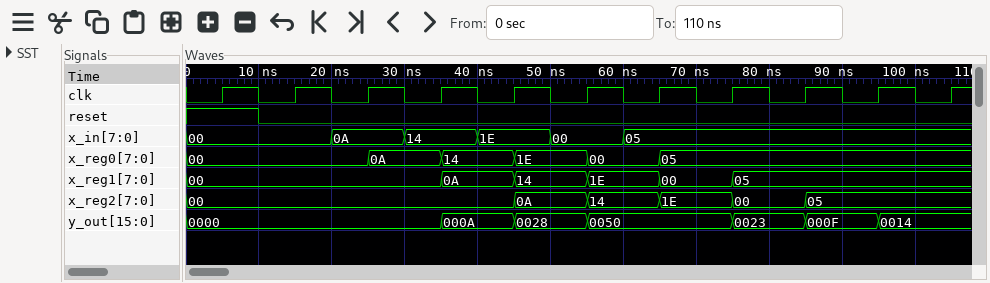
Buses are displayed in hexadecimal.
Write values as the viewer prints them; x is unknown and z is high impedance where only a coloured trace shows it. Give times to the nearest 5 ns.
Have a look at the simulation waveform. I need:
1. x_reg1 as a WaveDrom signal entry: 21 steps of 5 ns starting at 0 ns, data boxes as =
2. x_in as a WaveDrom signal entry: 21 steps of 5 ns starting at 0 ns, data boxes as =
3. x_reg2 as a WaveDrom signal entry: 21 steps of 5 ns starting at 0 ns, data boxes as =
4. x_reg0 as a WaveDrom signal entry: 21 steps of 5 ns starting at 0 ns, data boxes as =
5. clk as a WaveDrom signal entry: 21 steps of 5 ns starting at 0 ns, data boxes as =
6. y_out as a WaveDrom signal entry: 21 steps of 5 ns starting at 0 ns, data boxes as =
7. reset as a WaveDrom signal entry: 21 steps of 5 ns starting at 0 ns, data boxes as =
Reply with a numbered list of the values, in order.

1. {name: 'x_reg1', wave: '=......=.=.=.=.=.....', data: '00 0A 14 1E 00 05'}
2. {name: 'x_in', wave: '=...=.=.=.=.=........', data: '00 0A 14 1E 00 05'}
3. {name: 'x_reg2', wave: '=........=.=.=.=.=...', data: '00 0A 14 1E 00 05'}
4. {name: 'x_reg0', wave: '=....=.=.=.=.=.......', data: '00 0A 14 1E 00 05'}
5. {name: 'clk', wave: '010101010101010101010'}
6. {name: 'y_out', wave: '=......=.=.=...=.=.=.', data: '0000 000A 0028 0050 0023 000F 0014'}
7. {name: 'reset', wave: '1.0..................'}
